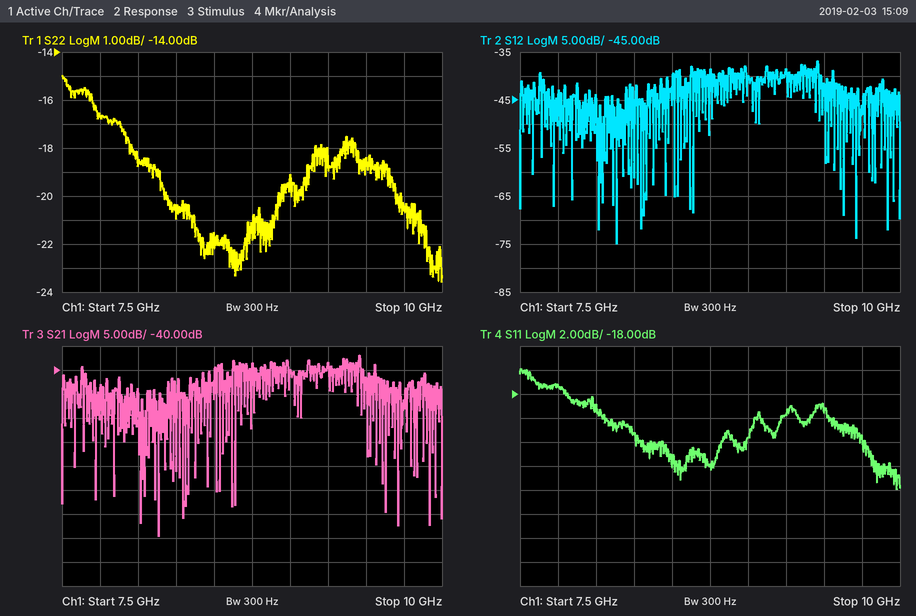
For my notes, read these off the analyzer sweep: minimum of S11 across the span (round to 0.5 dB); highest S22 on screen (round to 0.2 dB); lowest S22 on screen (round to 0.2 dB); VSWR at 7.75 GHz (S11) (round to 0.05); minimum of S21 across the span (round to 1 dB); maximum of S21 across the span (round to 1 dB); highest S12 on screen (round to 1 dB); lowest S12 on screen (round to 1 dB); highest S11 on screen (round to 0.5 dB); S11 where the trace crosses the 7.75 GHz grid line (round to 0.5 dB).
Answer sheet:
-26.0 dB
-15.0 dB
-23.6 dB
1.30
-75 dB
-37 dB
-37 dB
-75 dB
-16.0 dB
-17.5 dB
